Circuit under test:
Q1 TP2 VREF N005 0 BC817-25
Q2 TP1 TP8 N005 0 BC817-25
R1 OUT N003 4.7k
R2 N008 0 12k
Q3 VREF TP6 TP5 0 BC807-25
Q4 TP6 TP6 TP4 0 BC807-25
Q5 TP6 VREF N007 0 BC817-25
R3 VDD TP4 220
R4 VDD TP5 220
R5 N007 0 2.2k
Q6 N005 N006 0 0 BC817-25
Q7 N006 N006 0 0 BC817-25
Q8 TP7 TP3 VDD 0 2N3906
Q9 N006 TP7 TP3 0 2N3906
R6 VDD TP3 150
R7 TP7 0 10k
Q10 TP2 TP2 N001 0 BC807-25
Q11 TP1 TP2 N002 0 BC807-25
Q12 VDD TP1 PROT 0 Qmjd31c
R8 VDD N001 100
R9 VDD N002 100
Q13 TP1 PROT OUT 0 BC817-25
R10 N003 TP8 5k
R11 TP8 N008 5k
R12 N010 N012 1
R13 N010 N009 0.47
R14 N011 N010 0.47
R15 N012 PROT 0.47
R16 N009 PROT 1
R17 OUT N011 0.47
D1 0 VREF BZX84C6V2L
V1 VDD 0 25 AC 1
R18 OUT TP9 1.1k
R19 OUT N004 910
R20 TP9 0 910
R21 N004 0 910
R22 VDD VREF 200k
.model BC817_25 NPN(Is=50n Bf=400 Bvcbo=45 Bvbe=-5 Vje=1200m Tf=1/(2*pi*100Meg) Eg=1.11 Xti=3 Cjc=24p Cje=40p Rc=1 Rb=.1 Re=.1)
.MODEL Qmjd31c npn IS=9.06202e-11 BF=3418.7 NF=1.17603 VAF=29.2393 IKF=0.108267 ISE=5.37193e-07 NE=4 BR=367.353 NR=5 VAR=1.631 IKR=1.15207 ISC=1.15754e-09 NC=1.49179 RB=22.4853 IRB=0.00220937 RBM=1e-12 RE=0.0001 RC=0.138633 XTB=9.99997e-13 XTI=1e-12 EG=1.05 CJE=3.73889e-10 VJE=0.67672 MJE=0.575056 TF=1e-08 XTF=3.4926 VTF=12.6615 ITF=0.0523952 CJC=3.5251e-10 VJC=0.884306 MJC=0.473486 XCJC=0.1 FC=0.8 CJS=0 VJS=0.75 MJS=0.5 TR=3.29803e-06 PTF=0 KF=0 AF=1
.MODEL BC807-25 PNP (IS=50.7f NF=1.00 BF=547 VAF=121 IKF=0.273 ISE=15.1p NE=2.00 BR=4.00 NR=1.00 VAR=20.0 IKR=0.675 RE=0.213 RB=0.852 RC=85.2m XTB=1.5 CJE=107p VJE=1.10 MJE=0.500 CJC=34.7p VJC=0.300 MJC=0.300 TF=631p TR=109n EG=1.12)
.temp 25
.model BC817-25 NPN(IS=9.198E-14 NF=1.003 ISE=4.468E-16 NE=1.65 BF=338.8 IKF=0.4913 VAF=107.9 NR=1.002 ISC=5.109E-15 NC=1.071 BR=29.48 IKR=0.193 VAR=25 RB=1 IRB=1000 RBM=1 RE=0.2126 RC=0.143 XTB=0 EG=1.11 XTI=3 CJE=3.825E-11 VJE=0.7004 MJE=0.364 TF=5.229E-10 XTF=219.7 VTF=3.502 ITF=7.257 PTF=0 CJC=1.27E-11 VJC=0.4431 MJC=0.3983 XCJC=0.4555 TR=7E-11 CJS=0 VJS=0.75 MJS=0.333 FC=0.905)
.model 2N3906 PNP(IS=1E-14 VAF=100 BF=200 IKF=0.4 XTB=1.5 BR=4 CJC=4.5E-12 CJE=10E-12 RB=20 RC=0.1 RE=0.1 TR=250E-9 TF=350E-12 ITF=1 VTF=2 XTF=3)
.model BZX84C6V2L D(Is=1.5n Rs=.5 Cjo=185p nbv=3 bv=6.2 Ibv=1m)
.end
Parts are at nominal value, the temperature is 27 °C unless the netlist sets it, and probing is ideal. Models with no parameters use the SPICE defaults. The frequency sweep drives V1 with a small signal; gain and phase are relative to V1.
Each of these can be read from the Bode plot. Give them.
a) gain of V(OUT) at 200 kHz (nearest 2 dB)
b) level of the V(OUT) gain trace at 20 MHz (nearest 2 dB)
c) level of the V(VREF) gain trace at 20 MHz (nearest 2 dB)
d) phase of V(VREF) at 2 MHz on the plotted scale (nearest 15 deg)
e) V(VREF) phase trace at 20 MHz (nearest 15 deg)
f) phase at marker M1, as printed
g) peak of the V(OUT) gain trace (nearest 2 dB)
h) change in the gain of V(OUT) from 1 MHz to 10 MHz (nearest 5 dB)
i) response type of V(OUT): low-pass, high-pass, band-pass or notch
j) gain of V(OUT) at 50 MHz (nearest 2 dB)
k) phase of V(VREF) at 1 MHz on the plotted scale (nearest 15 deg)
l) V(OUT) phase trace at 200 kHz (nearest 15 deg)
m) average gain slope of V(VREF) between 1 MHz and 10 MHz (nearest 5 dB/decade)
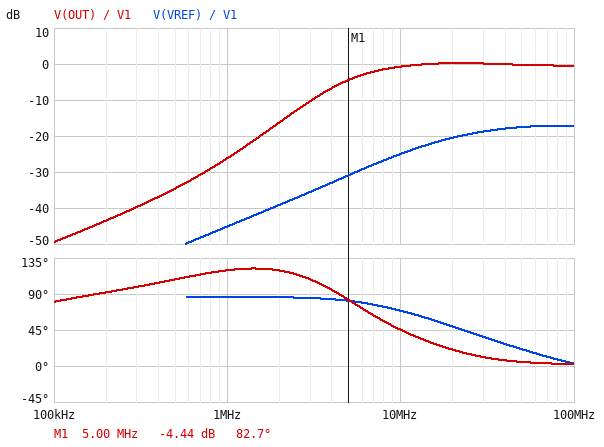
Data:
-44 dB
0 dB
-20 dB
90 deg
45 deg
82.7 deg
0 dB
25 dB
high-pass
0 dB
90 deg
90 deg
20 dB/decade
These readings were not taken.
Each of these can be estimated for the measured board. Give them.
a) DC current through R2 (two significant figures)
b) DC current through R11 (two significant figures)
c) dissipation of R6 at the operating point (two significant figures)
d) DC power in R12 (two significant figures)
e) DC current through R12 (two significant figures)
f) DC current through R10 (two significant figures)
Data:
370 µA
370 µA
3.1 mW
29 µW
5.4 mA
380 µA
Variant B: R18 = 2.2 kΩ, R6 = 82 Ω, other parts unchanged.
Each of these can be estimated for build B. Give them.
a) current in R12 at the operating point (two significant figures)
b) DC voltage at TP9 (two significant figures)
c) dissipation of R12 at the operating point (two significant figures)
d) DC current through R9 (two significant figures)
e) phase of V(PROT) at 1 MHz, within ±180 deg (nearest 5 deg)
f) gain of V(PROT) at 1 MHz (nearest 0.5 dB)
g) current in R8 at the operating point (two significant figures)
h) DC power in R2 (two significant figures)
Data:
4.5 mA
2.9 V
21 µW
4.4 mA
115 deg
-28.5 dB
4.3 mA
1.6 mW
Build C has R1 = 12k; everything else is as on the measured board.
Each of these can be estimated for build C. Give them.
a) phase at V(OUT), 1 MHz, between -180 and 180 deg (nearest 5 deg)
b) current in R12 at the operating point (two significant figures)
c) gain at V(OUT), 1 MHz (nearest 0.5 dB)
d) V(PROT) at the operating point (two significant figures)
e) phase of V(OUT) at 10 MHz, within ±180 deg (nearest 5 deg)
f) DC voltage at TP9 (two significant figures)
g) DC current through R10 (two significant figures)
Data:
115 deg
6.8 mA
-21.5 dB
13 V
35 deg
5.7 V
380 µA
